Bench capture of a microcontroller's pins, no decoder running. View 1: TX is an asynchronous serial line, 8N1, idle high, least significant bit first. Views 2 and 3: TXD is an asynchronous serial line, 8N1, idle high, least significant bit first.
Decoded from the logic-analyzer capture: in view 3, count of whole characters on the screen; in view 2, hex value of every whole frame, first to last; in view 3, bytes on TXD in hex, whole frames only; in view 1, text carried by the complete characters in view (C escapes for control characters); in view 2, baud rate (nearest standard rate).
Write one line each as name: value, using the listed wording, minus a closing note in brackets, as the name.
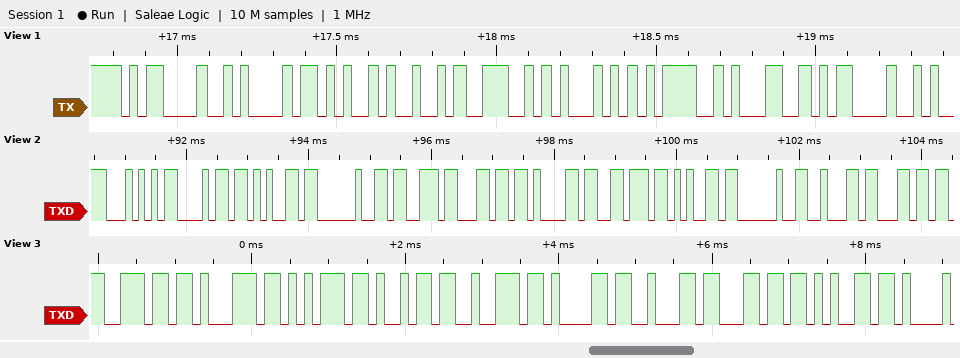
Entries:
in view 3, count of whole characters on the screen: 9
in view 2, hex value of every whole frame, first to last: 54 68 65 20 73 6C 61 76 65 20 62 6C
in view 3, bytes on TXD in hex, whole frames only: 6E 71 75 69 72 61 62 6C 65
in view 1, text carried by the complete characters in view: "\r\n+INQ=1\r"
in view 2, baud rate: 9600 baud
